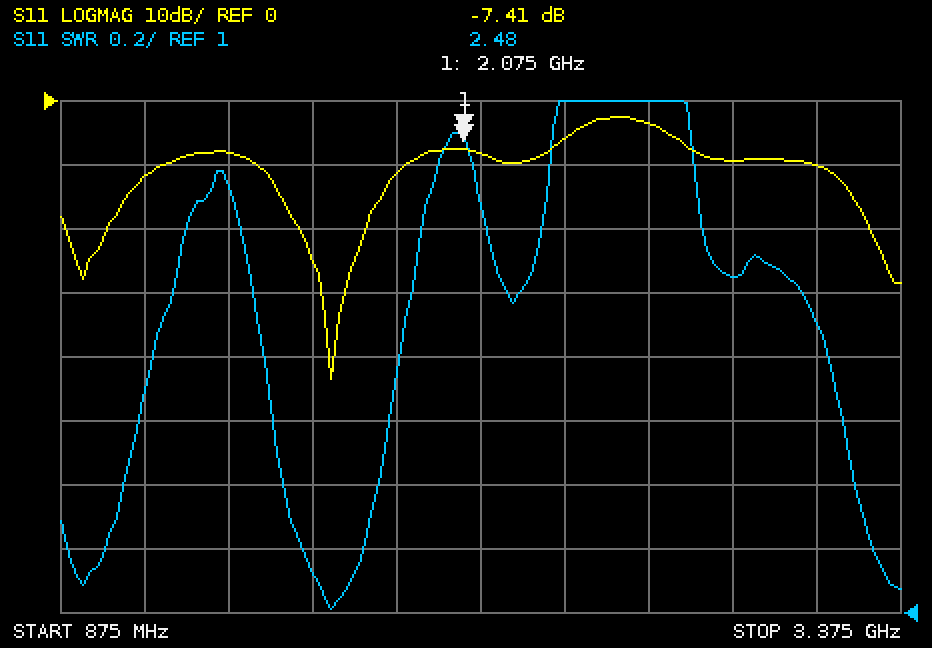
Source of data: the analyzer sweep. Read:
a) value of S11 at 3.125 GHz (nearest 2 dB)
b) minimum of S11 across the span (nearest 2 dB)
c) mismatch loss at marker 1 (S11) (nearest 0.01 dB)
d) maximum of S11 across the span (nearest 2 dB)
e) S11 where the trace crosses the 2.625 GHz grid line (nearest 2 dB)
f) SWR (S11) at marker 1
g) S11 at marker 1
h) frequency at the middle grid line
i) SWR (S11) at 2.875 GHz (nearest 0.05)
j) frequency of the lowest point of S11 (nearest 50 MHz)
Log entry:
-10 dB
-44 dB
0.87 dB
-2 dB
-4 dB
2.48
-7.41 dB
2.125 GHz
2.05
1.70 GHz
